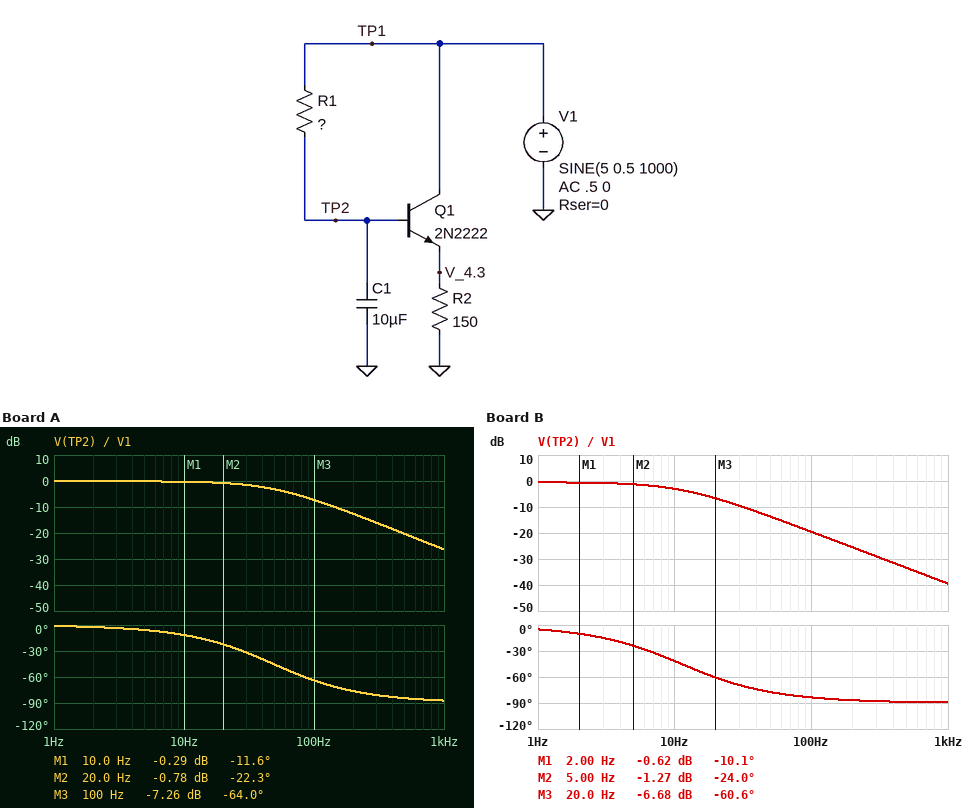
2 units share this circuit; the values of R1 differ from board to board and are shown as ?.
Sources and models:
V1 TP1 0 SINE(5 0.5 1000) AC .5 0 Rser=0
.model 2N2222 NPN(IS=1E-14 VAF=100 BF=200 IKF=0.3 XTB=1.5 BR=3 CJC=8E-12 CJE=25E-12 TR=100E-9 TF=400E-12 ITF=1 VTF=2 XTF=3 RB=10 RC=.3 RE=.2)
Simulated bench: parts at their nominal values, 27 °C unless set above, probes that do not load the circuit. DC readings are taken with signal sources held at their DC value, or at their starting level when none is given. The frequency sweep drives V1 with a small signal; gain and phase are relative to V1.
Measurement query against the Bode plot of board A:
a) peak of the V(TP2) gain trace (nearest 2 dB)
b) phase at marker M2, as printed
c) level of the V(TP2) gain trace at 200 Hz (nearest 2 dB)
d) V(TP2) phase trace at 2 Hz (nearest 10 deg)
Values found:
0 dB
-22.3 deg
-12 dB
0 deg
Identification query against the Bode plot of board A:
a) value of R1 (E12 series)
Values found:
330 Ω
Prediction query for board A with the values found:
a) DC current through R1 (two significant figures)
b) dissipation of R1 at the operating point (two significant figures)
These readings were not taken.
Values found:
150 µA
7.6 µW
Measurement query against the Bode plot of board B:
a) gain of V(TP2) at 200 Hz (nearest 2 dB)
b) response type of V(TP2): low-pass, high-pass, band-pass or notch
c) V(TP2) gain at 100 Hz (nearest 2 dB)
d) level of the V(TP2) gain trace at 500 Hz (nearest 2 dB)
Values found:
-26 dB
low-pass
-20 dB
-34 dB
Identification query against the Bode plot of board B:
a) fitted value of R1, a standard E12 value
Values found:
1.5 kΩ
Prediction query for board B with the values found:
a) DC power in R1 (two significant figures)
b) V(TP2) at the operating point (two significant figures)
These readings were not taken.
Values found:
32 µW
4.8 V
